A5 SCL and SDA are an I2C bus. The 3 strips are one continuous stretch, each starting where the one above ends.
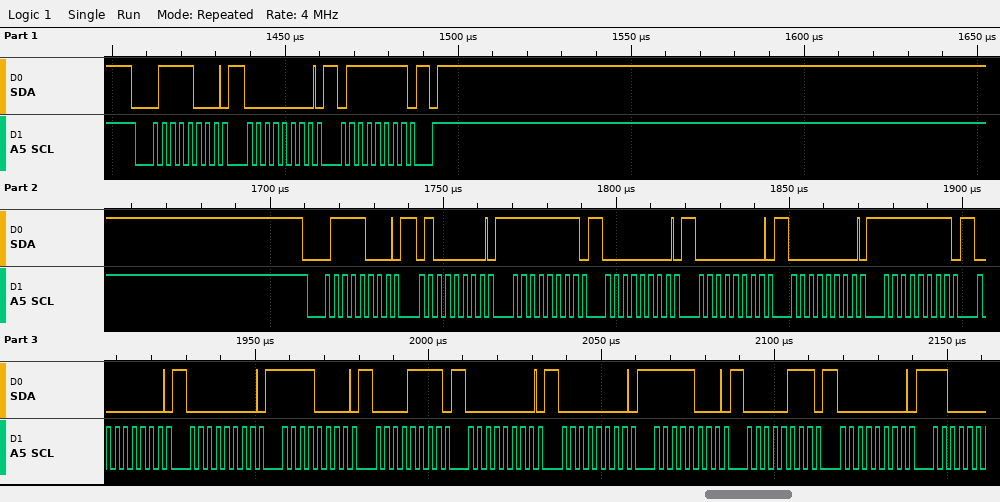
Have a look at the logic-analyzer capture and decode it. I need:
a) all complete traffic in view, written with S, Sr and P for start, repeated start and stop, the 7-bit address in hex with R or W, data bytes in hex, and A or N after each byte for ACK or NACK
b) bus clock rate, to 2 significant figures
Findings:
S 3CW A 00 A 7F A P S 3CW A 40 A FF A 00 A 00 A 00 A FF A 00 A 00 A F0 A 0F A 00 A 00 A F8 A 07 A 00 A
400 kHz
